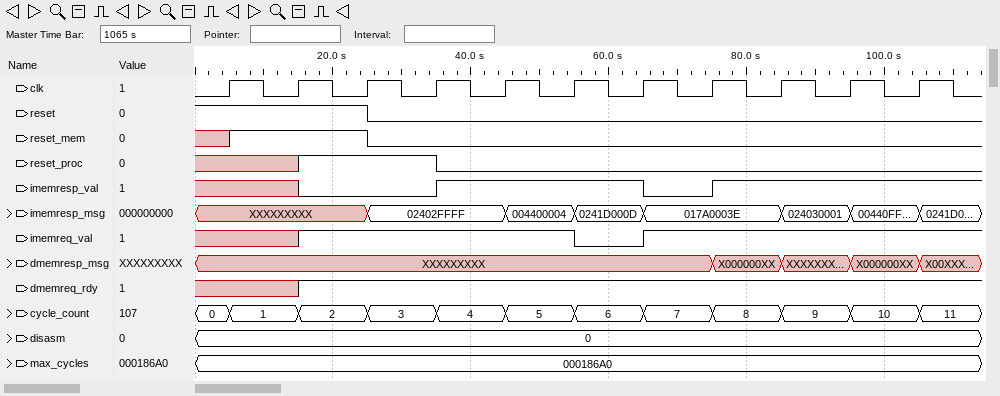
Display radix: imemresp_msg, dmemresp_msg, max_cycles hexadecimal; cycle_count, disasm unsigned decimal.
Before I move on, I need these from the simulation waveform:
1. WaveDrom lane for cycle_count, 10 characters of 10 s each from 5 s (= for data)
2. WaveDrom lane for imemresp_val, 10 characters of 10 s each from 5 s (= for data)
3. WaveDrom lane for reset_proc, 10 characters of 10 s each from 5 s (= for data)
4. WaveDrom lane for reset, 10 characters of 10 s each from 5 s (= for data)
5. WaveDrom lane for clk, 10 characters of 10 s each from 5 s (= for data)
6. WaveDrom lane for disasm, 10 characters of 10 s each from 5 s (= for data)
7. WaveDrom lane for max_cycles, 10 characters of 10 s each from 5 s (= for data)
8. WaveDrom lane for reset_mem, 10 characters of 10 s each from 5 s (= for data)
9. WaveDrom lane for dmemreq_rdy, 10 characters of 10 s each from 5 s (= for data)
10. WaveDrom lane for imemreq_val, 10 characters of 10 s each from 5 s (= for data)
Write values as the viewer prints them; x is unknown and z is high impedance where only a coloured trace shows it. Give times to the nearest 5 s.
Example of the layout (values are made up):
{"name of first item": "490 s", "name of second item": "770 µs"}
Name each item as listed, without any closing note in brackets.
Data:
{"WaveDrom lane for cycle_count, 10 characters of 10 s each from 5 s": "{name: 'cycle_count', wave: '==========', data: '1 2 3 4 5 6 7 8 9 10'}", "WaveDrom lane for imemresp_val, 10 characters of 10 s each from 5 s": "{name: 'imemresp_val', wave: 'x0.1..01..'}", "WaveDrom lane for reset_proc, 10 characters of 10 s each from 5 s": "{name: 'reset_proc', wave: 'x1.0......'}", "WaveDrom lane for reset, 10 characters of 10 s each from 5 s": "{name: 'reset', wave: '1.0.......'}", "WaveDrom lane for clk, 10 characters of 10 s each from 5 s": "{name: 'clk', wave: 'p.........'}", "WaveDrom lane for disasm, 10 characters of 10 s each from 5 s": "{name: 'disasm', wave: '=.........', data: '0'}", "WaveDrom lane for max_cycles, 10 characters of 10 s each from 5 s": "{name: 'max_cycles', wave: '=.........', data: '000186A0'}", "WaveDrom lane for reset_mem, 10 characters of 10 s each from 5 s": "{name: 'reset_mem', wave: '1.0.......'}", "WaveDrom lane for dmemreq_rdy, 10 characters of 10 s each from 5 s": "{name: 'dmemreq_rdy', wave: 'x1........'}", "WaveDrom lane for imemreq_val, 10 characters of 10 s each from 5 s": "{name: 'imemreq_val', wave: 'x1...01...'}"}
